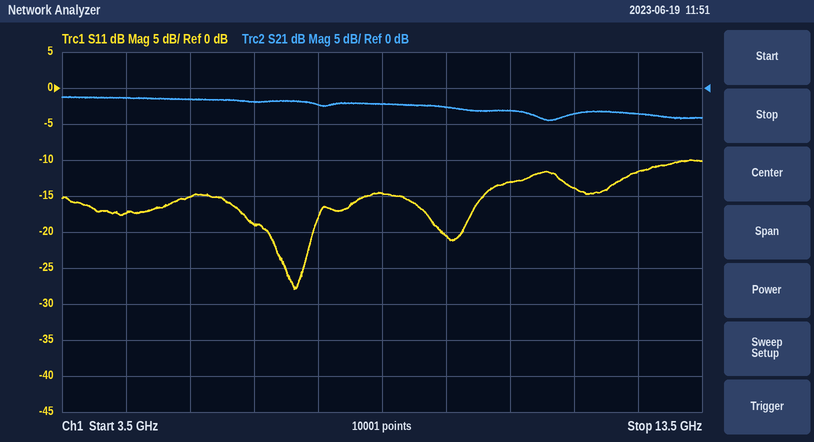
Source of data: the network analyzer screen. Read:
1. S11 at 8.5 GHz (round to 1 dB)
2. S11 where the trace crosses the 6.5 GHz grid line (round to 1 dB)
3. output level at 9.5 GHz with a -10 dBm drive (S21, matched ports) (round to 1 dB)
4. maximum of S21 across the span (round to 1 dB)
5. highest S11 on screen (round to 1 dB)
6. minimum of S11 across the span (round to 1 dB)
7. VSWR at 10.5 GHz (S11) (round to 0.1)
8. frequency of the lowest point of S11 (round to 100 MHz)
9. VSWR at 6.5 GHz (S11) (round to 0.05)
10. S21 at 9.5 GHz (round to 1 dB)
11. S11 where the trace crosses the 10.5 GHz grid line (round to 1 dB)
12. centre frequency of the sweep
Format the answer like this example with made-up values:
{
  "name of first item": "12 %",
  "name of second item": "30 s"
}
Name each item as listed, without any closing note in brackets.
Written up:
{
  "S11 at 8.5 GHz": "-15 dB",
  "S11 where the trace crosses the 6.5 GHz grid line": "-19 dB",
  "output level at 9.5 GHz with a -10 dBm drive (S21, matched ports)": "-13 dBm",
  "maximum of S21 across the span": "-1 dB",
  "highest S11 on screen": "-10 dB",
  "minimum of S11 across the span": "-28 dB",
  "VSWR at 10.5 GHz (S11)": "1.6",
  "frequency of the lowest point of S11": "7.1 GHz",
  "VSWR at 6.5 GHz (S11)": "1.25",
  "S21 at 9.5 GHz": "-3 dB",
  "S11 where the trace crosses the 10.5 GHz grid line": "-13 dB",
  "centre frequency of the sweep": "8.5 GHz"
}
